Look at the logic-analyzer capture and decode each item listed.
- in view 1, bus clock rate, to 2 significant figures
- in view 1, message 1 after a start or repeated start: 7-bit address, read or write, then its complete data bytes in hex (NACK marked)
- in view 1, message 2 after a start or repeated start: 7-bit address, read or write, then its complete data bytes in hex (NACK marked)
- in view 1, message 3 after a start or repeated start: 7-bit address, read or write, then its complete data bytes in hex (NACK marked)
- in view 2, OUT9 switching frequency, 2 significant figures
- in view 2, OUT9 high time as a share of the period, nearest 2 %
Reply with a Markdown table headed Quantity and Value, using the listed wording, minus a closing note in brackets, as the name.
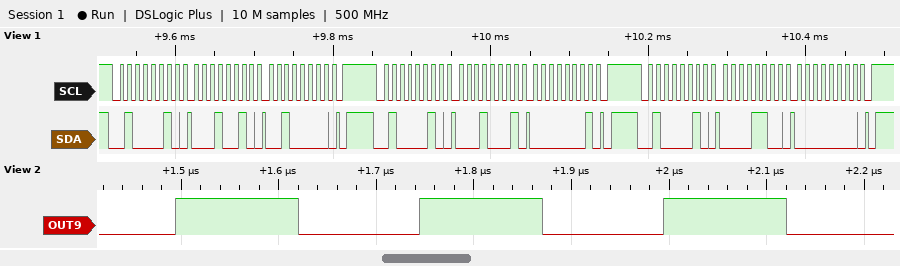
| Quantity | Value |
|---|---|
| in view 1, bus clock rate, to 2 significant figures | 100 kHz |
| in view 1, message 1 after a start or repeated start: 7-bit address, read or write, then its complete data bytes in hex | 0x21 write: 12 20 |
| in view 1, message 2 after a start or repeated start: 7-bit address, read or write, then its complete data bytes in hex | 0x21 write: 11 01 |
| in view 1, message 3 after a start or repeated start: 7-bit address, read or write, then its complete data bytes in hex | 0x21 write: 0C 00 |
| in view 2, OUT9 switching frequency, 2 significant figures | 4.0 MHz |
| in view 2, OUT9 high time as a share of the period, nearest 2 % | 50 % |
